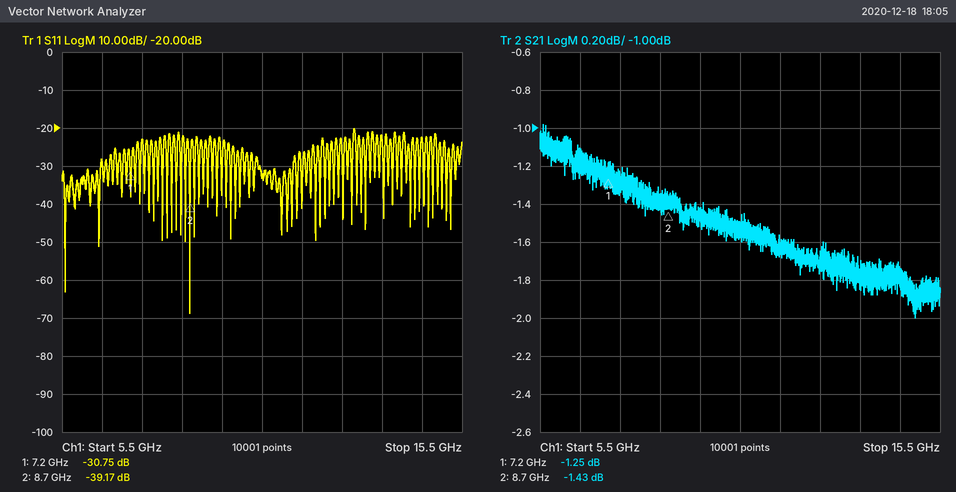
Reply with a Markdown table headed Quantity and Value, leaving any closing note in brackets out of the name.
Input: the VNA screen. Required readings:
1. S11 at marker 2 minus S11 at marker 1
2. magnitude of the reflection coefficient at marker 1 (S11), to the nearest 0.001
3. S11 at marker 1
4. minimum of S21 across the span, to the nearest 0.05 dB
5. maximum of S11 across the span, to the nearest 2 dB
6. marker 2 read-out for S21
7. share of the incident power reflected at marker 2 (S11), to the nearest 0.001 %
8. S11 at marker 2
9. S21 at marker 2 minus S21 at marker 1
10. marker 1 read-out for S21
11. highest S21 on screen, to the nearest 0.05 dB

| Quantity | Value |
|---|---|
| S11 at marker 2 minus S11 at marker 1 | -8.42 dB |
| magnitude of the reflection coefficient at marker 1 (S11), to the nearest 0.001 | 0.029 |
| S11 at marker 1 | -30.75 dB |
| minimum of S21 across the span, to the nearest 0.05 dB | -2.00 dB |
| maximum of S11 across the span, to the nearest 2 dB | -20 dB |
| marker 2 read-out for S21 | -1.43 dB |
| share of the incident power reflected at marker 2 (S11), to the nearest 0.001 % | 0.012 % |
| S11 at marker 2 | -39.17 dB |
| S21 at marker 2 minus S21 at marker 1 | -0.18 dB |
| marker 1 read-out for S21 | -1.25 dB |
| highest S21 on screen, to the nearest 0.05 dB | -1.00 dB |
